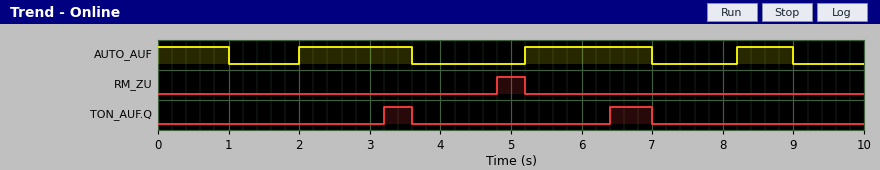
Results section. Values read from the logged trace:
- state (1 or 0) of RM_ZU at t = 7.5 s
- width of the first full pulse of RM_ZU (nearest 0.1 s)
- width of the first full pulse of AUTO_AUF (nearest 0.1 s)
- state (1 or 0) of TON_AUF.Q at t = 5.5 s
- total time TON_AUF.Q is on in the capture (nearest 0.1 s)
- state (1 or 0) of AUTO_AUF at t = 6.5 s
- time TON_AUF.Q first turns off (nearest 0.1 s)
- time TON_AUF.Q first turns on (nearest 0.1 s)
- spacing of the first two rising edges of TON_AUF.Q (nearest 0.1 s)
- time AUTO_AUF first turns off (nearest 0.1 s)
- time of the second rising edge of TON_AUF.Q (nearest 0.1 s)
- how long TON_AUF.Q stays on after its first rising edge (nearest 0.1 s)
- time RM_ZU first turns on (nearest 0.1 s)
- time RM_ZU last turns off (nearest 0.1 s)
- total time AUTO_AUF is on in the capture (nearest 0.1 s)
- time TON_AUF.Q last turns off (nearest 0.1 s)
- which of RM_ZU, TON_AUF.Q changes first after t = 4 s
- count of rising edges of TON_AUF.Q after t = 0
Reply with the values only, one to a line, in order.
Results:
0
0.4 s
1.6 s
0
1.0 s
1
3.6 s
3.2 s
3.2 s
1.0 s
6.4 s
0.4 s
4.8 s
5.2 s
5.2 s
7.0 s
RM_ZU
2
